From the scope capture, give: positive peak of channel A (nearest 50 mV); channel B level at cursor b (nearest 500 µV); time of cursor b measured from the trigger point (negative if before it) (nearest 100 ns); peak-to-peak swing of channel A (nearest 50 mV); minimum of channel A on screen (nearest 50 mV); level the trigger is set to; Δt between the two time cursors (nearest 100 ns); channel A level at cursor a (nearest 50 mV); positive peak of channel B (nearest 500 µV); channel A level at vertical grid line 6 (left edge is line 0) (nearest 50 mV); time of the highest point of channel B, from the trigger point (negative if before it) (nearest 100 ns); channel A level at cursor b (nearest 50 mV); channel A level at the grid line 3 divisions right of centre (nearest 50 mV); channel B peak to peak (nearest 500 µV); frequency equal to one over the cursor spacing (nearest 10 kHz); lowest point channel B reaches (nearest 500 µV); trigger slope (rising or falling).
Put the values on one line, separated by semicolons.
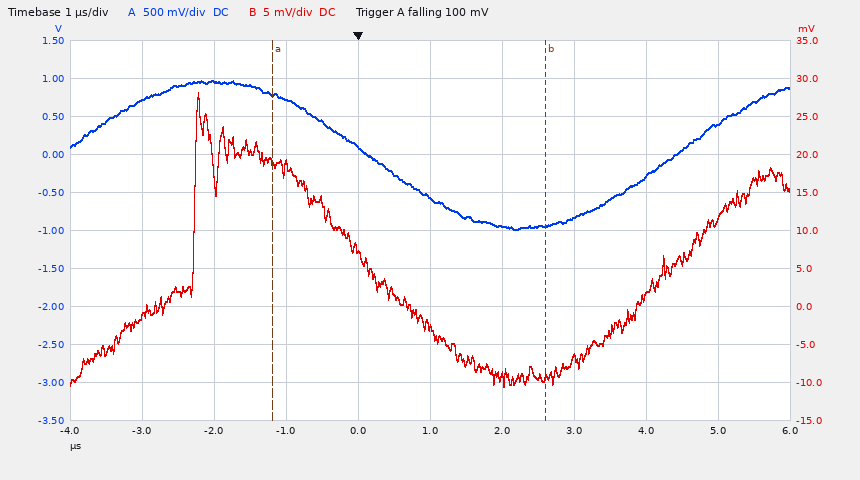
950 mV; -9.5 mV; +2.6 µs; 1.95 V; -1.00 V; 100 mV; 3.8 µs; 800 mV; 28.0 mV; -950 mV; -2.2 µs; -950 mV; -300 mV; 38.5 mV; 260 kHz; -10.5 mV; falling
